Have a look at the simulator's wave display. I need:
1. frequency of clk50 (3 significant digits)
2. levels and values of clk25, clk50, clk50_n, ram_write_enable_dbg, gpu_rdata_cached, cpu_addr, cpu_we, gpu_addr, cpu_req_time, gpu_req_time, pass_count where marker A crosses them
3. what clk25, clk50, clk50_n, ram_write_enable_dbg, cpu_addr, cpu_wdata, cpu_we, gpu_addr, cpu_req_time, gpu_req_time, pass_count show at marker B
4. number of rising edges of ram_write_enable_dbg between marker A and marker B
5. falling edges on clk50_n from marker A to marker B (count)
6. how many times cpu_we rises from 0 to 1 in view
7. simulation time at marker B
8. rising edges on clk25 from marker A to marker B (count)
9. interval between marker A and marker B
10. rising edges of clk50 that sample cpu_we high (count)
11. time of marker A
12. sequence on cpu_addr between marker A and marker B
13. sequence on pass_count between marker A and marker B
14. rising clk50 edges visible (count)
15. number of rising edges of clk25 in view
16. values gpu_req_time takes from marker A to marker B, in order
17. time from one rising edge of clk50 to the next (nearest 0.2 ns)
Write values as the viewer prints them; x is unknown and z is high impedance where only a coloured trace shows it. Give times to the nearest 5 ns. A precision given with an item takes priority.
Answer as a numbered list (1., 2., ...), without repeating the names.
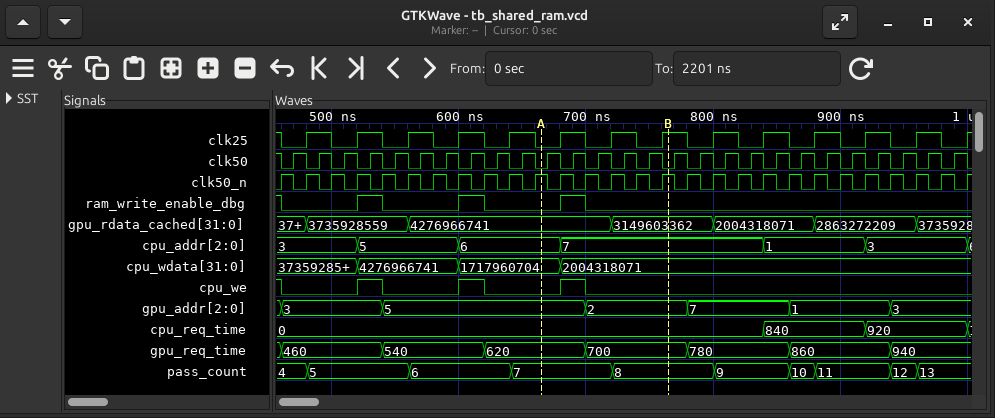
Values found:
1. 50.0 MHz
2. clk25=0, clk50=0, clk50_n=1, ram_write_enable_dbg=0, gpu_rdata_cached=4276966741, cpu_addr=6, cpu_we=0, gpu_addr=5, cpu_req_time=0, gpu_req_time=620, pass_count=7
3. clk25=1, clk50=0, clk50_n=1, ram_write_enable_dbg=0, cpu_addr=7, cpu_wdata=2004318071, cpu_we=0, gpu_addr=2, cpu_req_time=0, gpu_req_time=700, pass_count=8
4. 1
5. 5
6. 3
7. 765 ns
8. 3
9. 100 ns
10. 3
11. 665 ns
12. 6, 7
13. 7, 8
14. 27
15. 14
16. 620, 700
17. 20 ns
